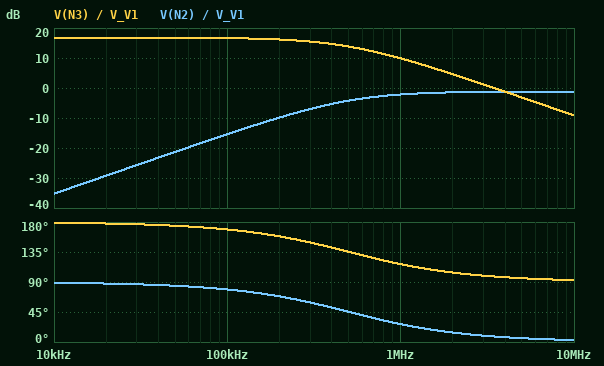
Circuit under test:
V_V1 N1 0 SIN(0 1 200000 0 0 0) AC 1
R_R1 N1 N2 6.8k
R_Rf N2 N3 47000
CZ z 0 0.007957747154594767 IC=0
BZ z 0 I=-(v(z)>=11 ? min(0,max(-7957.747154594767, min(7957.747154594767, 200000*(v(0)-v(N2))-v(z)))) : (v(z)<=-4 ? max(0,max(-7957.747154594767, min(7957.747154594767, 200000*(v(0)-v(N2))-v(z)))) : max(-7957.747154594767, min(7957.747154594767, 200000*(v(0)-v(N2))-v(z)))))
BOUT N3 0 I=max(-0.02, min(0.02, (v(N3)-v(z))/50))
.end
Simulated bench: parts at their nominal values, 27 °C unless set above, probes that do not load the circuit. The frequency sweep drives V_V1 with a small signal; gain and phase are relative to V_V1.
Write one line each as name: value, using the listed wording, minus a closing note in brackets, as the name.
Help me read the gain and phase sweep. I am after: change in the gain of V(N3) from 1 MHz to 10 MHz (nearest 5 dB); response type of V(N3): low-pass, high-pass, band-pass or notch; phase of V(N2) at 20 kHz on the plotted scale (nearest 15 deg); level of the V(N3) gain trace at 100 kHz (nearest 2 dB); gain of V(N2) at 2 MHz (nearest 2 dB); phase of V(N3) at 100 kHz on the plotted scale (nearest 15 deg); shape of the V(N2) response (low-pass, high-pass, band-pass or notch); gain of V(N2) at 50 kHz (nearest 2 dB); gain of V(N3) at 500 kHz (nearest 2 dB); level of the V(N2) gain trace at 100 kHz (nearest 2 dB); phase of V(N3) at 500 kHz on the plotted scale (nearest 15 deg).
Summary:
change in the gain of V(N3) from 1 MHz to 10 MHz: -20 dB
response type of V(N3): low-pass, high-pass, band-pass or notch: low-pass
phase of V(N2) at 20 kHz on the plotted scale: 90 deg
level of the V(N3) gain trace at 100 kHz: 16 dB
gain of V(N2) at 2 MHz: -2 dB
phase of V(N3) at 100 kHz on the plotted scale: 165 deg
shape of the V(N2) response: high-pass
gain of V(N2) at 50 kHz: -22 dB
gain of V(N3) at 500 kHz: 14 dB
level of the V(N2) gain trace at 100 kHz: -16 dB
phase of V(N3) at 500 kHz on the plotted scale: 135 deg
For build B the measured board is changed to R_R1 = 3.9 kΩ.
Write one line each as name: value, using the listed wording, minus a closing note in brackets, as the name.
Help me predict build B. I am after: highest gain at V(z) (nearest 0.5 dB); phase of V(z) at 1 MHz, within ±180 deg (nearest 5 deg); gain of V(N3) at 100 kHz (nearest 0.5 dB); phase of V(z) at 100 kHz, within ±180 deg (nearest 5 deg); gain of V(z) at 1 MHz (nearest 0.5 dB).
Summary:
highest gain at V(z): 21.5 dB
phase of V(z) at 1 MHz, within ±180 deg: 105 deg
gain of V(N3) at 100 kHz: 21.0 dB
phase of V(z) at 100 kHz, within ±180 deg: 160 deg
gain of V(z) at 1 MHz: 11.0 dB
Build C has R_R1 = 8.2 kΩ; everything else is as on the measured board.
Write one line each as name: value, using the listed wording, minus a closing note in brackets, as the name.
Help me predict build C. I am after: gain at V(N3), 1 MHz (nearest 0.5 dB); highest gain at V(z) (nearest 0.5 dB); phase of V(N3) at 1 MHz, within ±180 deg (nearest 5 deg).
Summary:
gain at V(N3), 1 MHz: 9.5 dB
highest gain at V(z): 15.0 dB
phase of V(N3) at 1 MHz, within ±180 deg: 120 deg
